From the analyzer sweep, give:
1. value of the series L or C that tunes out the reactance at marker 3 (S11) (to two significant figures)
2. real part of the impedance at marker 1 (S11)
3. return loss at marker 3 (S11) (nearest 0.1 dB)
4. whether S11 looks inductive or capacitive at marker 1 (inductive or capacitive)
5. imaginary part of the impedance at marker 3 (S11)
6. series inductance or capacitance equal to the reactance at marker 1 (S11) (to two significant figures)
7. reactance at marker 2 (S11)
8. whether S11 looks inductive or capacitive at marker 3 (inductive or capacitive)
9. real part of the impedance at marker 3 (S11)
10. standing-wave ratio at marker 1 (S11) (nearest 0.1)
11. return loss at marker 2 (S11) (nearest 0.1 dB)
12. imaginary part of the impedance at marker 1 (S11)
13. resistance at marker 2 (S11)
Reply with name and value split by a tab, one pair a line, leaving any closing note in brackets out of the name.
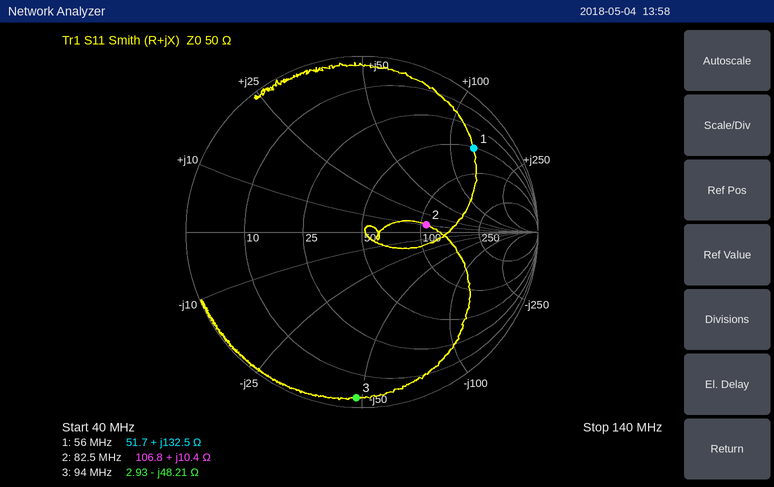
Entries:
value of the series L or C that tunes out the reactance at marker 3 (S11)	82 nH
real part of the impedance at marker 1	51.7 Ω
return loss at marker 3 (S11)	0.5 dB
whether S11 looks inductive or capacitive at marker 1	inductive
imaginary part of the impedance at marker 3	-48.21 Ω
series inductance or capacitance equal to the reactance at marker 1 (S11)	380 nH
reactance at marker 2	+10.4 Ω
whether S11 looks inductive or capacitive at marker 3	capacitive
real part of the impedance at marker 3	2.93 Ω
standing-wave ratio at marker 1 (S11)	8.7
return loss at marker 2 (S11)	8.7 dB
imaginary part of the impedance at marker 1	+132.5 Ω
resistance at marker 2	106.8 Ω
